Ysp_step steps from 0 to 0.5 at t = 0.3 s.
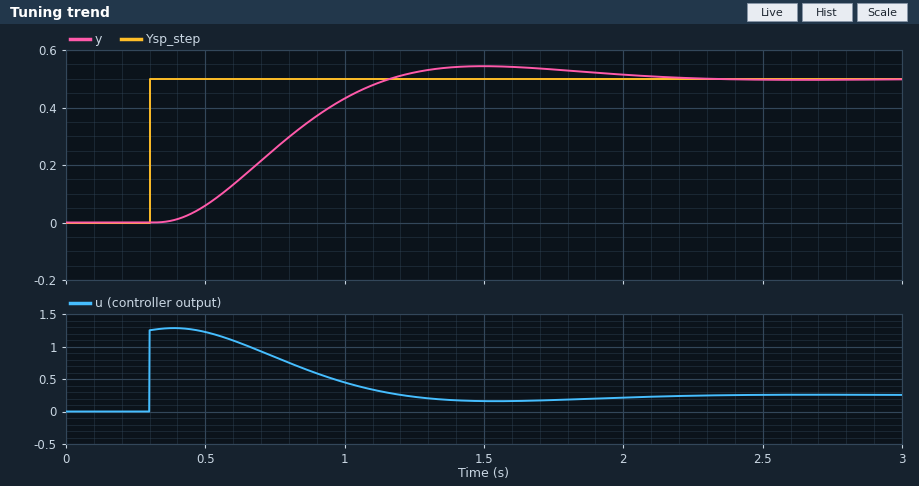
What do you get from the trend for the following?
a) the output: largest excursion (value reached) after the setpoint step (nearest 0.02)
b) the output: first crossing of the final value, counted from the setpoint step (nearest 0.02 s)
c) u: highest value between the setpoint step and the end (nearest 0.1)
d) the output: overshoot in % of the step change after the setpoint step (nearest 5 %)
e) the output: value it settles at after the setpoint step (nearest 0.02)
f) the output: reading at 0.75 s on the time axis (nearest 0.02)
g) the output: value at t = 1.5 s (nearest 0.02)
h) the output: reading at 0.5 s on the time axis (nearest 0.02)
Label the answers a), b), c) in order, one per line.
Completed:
a) 0.54
b) 0.86 s
c) 1.3
d) 10 %
e) 0.50
f) 0.26
g) 0.54
h) 0.06
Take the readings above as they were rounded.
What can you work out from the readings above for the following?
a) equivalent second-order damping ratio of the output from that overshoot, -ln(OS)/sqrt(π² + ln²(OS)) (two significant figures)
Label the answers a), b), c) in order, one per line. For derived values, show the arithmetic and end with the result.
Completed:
a) ln(0.1) = -2.303; 2.303 / sqrt(9.870 + 5.302) = 0.59
